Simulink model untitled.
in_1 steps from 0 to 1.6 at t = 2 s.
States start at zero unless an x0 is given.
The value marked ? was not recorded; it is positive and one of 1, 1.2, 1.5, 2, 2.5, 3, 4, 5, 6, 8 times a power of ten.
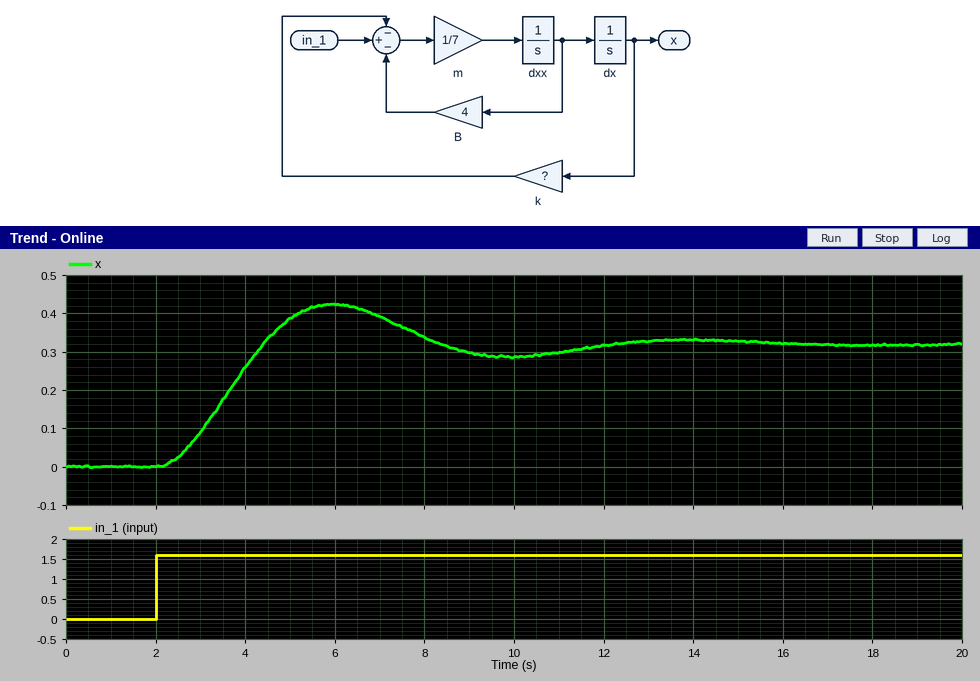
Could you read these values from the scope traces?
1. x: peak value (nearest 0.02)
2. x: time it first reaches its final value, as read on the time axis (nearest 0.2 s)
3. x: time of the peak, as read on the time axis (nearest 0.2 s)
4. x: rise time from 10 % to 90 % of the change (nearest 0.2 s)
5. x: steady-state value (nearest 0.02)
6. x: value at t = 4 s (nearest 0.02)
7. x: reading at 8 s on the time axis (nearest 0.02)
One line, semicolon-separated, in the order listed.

0.42; 4.4 s; 6.0 s; 1.6 s; 0.32; 0.26; 0.34
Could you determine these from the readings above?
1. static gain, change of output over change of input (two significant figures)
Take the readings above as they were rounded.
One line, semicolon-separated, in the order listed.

0.20
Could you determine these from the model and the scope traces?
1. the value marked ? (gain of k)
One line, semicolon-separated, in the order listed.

5
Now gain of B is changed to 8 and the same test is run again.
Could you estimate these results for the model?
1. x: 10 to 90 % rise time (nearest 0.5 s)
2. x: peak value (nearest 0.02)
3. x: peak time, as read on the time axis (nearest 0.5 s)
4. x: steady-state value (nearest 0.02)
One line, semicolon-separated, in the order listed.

2.5 s; 0.34; 7.0 s; 0.32
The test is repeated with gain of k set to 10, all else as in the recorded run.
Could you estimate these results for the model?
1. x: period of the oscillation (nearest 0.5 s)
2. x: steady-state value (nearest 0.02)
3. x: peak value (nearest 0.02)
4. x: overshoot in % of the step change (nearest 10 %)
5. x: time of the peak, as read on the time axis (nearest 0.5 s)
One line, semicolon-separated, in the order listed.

5.5 s; 0.16; 0.24; 50 %; 4.5 s
